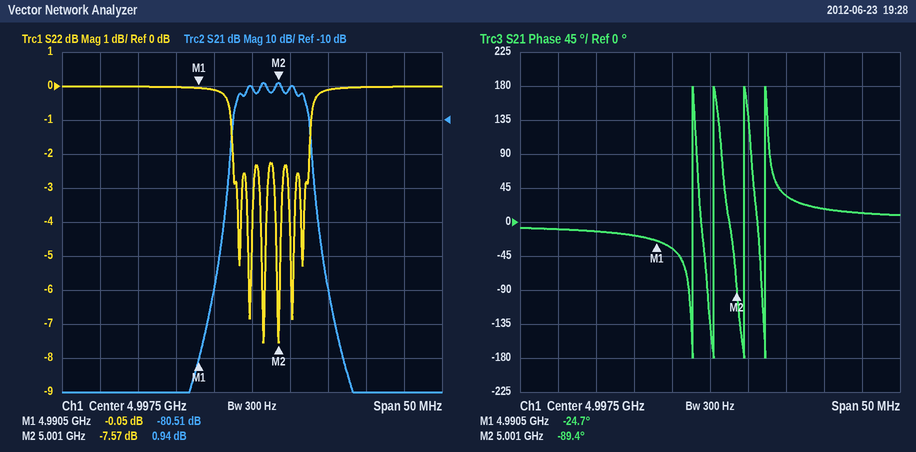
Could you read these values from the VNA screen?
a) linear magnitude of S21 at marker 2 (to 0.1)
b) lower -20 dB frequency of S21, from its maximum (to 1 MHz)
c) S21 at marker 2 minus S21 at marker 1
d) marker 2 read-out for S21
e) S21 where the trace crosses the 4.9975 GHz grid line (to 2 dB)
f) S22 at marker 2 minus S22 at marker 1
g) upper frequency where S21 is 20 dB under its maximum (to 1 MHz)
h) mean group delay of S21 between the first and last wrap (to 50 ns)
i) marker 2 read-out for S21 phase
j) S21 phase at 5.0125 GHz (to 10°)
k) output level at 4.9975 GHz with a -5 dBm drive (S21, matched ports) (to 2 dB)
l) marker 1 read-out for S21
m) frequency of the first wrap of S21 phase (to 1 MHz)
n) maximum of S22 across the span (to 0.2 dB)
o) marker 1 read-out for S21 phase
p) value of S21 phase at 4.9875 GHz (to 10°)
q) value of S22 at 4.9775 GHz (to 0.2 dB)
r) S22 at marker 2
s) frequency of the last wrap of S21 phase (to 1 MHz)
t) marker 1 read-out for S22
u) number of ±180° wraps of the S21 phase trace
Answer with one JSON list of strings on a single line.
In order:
["1.1", "4.995 GHz", "81.45 dB", "0.94 dB", "0 dB", "-7.52 dB", "5.005 GHz", "300 ns", "-89.4°", "20°", "-6 dBm", "-80.51 dB", "4.995 GHz", "0.0 dB", "-24.7°", "-20°", "0.0 dB", "-7.57 dB", "5.005 GHz", "-0.05 dB", "4"]
